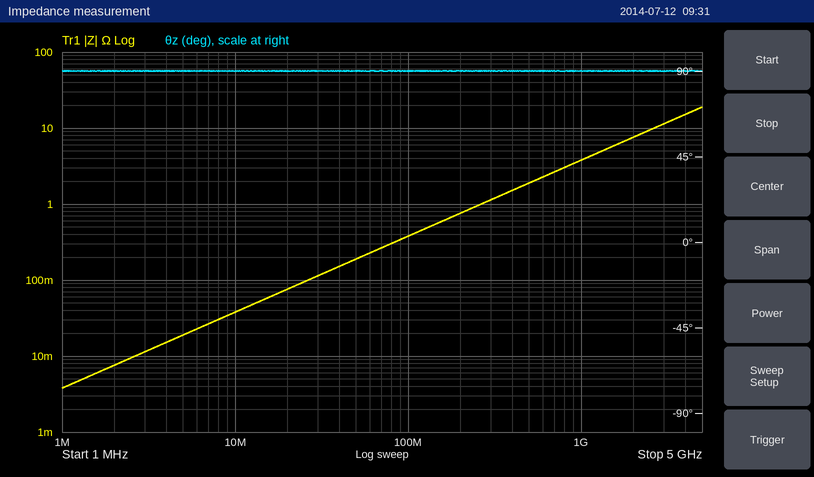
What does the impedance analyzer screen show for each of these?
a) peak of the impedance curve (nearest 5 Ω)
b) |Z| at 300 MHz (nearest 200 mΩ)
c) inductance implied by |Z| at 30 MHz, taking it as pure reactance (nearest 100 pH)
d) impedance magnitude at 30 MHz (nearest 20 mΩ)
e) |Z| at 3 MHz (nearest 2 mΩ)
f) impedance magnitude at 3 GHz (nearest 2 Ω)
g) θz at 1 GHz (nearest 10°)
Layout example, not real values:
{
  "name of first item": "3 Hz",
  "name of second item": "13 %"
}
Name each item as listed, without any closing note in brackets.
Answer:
{
  "peak of the impedance curve": "20 Ω",
  "|Z| at 300 MHz": "1.2 Ω",
  "inductance implied by |Z| at 30 MHz, taking it as pure reactance": "600 pH",
  "impedance magnitude at 30 MHz": "120 mΩ",
  "|Z| at 3 MHz": "12 mΩ",
  "impedance magnitude at 3 GHz": "12 Ω",
  "θz at 1 GHz": "90°"
}
